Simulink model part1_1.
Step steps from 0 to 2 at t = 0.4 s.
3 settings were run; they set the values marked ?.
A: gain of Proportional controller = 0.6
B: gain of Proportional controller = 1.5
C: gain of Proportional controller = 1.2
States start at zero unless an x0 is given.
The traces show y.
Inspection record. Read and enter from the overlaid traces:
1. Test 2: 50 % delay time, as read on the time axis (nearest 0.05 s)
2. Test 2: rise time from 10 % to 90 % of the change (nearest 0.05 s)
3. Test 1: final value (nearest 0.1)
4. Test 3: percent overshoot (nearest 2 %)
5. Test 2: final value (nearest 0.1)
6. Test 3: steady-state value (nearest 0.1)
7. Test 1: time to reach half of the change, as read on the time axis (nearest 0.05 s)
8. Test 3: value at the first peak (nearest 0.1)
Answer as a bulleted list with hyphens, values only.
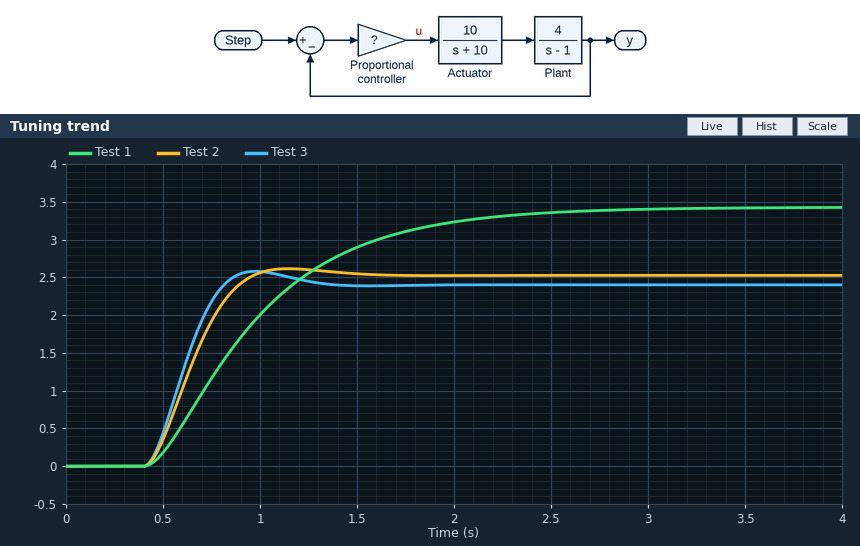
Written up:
- 0.65 s
- 0.35 s
- 3.4
- 8 %
- 2.5
- 2.4
- 0.90 s
- 2.6
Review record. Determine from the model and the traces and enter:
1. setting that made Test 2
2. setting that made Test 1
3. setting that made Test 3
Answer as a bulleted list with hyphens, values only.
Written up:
- C
- A
- B
